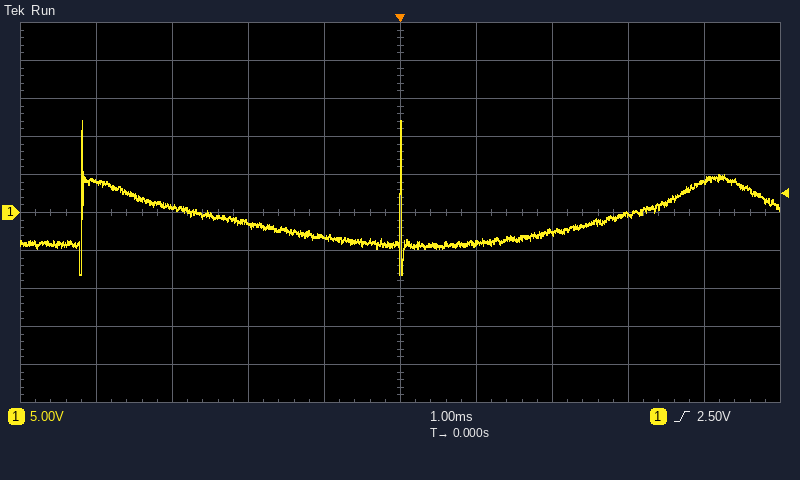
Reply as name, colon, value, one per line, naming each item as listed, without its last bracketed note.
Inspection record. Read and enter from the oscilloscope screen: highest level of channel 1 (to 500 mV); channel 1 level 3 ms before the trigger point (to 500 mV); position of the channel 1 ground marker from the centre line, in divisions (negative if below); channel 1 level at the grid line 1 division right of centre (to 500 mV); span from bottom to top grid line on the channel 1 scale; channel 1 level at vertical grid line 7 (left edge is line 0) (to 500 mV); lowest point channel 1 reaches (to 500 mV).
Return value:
highest level of channel 1: 12.0 V
channel 1 level 3 ms before the trigger point: 1.0 V
position of the channel 1 ground marker from the centre line, in divisions: 0.0 div
channel 1 level at the grid line 1 division right of centre: -4.0 V
span from bottom to top grid line on the channel 1 scale: 50 V
channel 1 level at vertical grid line 7 (left edge is line 0): -2.5 V
lowest point channel 1 reaches: -8.0 V
